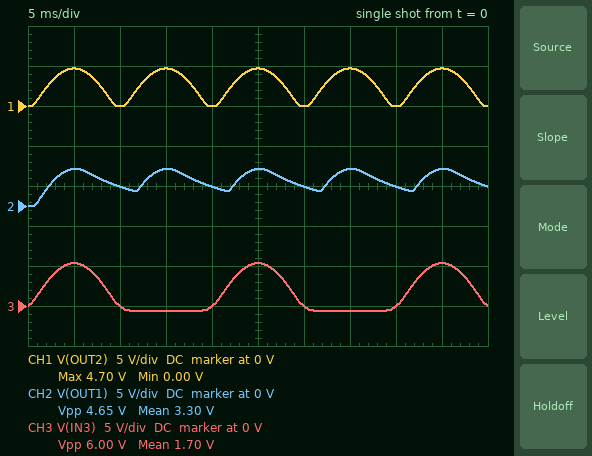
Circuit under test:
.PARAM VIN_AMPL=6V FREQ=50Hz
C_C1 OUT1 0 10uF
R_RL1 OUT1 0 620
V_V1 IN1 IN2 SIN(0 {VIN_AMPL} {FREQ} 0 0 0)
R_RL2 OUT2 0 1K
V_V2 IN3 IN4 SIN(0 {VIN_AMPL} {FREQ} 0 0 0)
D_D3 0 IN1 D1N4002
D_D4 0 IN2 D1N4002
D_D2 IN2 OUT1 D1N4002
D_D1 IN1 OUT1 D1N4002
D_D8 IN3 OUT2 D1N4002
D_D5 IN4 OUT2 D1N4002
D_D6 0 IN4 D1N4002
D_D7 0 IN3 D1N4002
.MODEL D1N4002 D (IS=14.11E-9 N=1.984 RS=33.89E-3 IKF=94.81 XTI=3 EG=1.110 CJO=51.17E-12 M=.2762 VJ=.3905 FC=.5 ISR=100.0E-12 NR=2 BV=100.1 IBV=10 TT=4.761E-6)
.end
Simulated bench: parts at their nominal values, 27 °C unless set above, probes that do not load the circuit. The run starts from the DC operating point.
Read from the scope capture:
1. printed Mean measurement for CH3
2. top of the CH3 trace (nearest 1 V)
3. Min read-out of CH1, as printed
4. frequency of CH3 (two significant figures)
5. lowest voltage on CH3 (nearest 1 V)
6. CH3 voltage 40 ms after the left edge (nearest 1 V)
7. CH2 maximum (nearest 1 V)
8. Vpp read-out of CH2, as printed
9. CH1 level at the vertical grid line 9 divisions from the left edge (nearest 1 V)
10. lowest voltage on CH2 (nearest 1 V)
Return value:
1.70 V
5 V
0.00 V
50 Hz
-1 V
0 V
5 V
4.65 V
5 V
0 V
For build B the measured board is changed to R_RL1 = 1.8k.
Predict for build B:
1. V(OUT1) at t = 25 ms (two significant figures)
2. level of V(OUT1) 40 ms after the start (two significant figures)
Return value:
4.7 V
3.7 V
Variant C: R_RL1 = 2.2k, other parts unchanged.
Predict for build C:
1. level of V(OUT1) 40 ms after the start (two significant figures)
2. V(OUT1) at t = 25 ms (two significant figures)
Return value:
3.9 V
4.7 V
